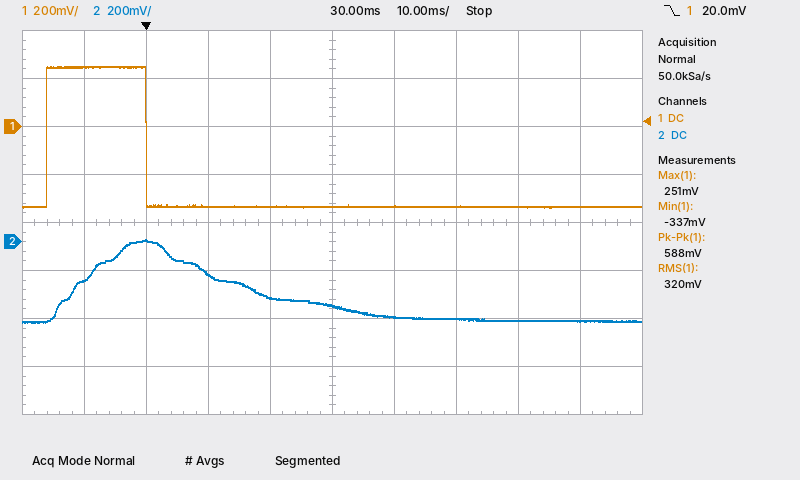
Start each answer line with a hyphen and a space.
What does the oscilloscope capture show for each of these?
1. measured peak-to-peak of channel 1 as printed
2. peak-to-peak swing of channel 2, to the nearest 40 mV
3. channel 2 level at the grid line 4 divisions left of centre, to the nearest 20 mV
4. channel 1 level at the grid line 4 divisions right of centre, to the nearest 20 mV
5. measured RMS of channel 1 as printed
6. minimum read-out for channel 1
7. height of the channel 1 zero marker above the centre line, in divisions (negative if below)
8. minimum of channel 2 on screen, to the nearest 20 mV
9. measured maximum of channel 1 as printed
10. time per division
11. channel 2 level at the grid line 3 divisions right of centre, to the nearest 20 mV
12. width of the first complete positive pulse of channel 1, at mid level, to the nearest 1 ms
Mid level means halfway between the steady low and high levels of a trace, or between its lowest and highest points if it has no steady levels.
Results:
- 588 mV
- 360 mV
- -160 mV
- -340 mV
- 320 mV
- -337 mV
- +2.0 div
- -340 mV
- 251 mV
- 10 ms
- -320 mV
- 16 ms
